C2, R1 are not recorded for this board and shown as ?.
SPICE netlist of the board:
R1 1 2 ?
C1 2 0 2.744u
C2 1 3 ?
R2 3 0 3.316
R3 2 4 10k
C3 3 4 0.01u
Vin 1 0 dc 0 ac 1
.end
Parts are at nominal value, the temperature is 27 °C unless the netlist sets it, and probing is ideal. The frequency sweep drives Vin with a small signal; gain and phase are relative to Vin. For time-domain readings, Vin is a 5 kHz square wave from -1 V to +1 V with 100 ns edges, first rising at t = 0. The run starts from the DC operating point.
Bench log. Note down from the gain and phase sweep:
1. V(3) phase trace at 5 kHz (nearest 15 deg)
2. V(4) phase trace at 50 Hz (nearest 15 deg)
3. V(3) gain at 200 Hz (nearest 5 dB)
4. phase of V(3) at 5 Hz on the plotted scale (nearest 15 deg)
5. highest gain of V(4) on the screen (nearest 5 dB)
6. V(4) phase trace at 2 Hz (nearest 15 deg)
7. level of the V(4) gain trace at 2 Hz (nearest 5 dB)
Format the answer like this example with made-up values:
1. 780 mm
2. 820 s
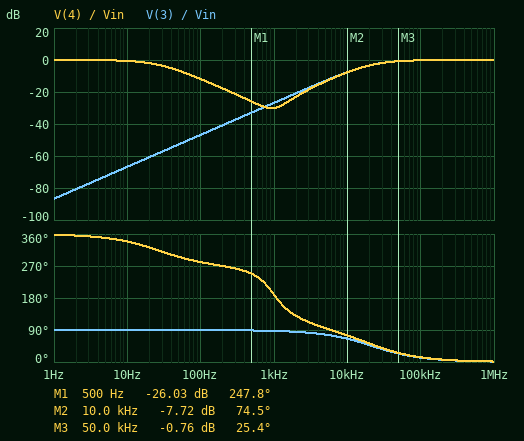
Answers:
1. 75 deg
2. 300 deg
3. -40 dB
4. 90 deg
5. 0 dB
6. 360 deg
7. 0 dB
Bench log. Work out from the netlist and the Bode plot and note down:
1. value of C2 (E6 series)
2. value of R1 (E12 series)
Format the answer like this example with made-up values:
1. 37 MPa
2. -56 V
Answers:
1. 2.2 µF
2. 2.2 kΩ
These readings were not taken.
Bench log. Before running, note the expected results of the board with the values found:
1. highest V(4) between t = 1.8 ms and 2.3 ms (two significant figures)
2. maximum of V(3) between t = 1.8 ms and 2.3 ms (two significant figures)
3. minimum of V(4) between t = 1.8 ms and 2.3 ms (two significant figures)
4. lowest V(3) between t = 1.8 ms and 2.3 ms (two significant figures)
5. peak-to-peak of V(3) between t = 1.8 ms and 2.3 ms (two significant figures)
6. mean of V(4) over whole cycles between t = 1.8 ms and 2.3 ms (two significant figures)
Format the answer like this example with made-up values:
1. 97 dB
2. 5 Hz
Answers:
1. 1.3 V
2. 2.0 V
3. -2.8 V
4. -2.0 V
5. 4.0 V
6. -730 mV
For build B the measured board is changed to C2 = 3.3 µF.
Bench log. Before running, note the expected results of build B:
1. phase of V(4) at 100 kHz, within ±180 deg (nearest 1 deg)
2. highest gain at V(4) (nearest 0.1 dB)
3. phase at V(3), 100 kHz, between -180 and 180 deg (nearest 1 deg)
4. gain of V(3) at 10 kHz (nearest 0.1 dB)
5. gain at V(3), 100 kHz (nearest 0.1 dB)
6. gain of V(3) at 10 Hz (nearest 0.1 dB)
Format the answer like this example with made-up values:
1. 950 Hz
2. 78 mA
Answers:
1. 9 deg
2. 0 dB
3. 8 deg
4. -4.9 dB
5. -0.1 dB
6. -63.2 dB
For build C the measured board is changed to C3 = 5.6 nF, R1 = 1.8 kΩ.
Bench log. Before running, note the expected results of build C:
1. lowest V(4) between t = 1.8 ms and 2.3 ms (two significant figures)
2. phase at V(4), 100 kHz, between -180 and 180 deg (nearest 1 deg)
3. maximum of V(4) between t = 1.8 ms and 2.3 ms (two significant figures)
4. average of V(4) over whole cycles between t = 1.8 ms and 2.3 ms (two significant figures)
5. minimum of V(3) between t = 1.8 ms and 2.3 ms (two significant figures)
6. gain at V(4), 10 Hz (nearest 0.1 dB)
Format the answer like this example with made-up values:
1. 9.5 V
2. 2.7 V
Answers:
1. -2.7 V
2. 14 deg
3. 1.4 V
4. -670 mV
5. -2.0 V
6. -0.4 dB
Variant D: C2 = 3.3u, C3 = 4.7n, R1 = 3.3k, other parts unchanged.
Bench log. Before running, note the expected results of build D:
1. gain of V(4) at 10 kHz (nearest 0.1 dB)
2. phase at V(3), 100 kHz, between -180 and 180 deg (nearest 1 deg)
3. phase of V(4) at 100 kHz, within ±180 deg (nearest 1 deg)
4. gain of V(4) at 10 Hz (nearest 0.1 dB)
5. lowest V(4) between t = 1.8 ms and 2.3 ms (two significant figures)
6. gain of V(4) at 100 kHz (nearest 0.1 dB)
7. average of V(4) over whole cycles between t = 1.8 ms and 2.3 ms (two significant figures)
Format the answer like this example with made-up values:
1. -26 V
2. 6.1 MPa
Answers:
1. -5.4 dB
2. 8 deg
3. 10 deg
4. -1.2 dB
5. -2.9 V
6. -0.1 dB
7. -800 mV
